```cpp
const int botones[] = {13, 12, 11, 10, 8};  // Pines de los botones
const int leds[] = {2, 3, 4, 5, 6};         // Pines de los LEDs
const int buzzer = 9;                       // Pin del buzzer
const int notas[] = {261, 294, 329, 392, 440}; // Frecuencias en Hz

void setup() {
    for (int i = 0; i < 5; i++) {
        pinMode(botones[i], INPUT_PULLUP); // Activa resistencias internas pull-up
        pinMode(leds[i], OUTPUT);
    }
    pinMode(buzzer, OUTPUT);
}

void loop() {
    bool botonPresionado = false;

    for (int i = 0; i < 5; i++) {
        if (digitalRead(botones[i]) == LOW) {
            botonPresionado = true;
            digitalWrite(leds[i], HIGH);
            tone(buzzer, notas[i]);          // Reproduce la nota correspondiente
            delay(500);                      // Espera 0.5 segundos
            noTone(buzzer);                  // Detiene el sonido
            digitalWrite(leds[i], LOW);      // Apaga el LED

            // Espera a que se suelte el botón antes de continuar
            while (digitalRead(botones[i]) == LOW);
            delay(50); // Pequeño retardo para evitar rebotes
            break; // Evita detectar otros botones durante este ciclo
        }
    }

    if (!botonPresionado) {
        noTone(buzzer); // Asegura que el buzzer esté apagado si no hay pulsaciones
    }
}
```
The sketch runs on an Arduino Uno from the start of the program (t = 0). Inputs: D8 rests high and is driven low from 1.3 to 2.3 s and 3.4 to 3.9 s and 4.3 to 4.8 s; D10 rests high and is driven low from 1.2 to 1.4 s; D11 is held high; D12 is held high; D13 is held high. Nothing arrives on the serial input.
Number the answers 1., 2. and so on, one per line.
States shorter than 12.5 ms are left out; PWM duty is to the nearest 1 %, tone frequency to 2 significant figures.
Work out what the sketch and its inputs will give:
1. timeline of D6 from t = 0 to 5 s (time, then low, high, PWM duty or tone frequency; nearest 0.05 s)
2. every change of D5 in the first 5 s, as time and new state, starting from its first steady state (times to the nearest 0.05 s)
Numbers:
1. 0 s low; 1.75 s high; 2.25 s low; 3.4 s high; 3.9 s low; 4.3 s high; 4.8 s low
2. 0 s low; 1.2 s high; 1.7 s low
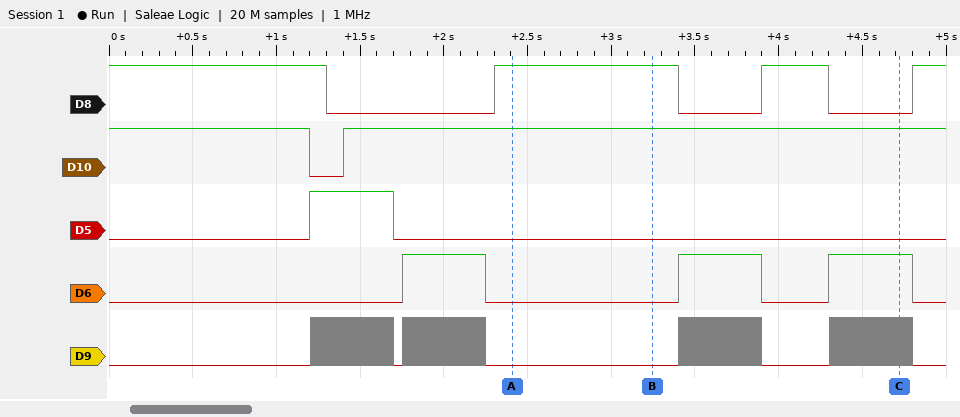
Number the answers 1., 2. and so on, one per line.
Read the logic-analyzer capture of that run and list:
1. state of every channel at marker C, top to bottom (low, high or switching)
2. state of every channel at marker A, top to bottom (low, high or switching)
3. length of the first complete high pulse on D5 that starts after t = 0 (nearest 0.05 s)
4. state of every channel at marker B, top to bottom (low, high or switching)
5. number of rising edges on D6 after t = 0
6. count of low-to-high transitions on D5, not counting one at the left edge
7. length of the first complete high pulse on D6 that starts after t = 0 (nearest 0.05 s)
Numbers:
1. D8 low, D10 high, D5 low, D6 high, D9 switching
2. D8 high, D10 high, D5 low, D6 low, D9 low
3. 0.50 s
4. D8 high, D10 high, D5 low, D6 low, D9 low
5. 3
6. 1
7. 0.50 s
